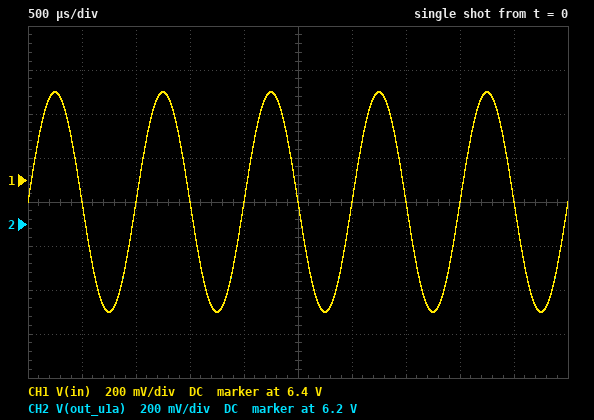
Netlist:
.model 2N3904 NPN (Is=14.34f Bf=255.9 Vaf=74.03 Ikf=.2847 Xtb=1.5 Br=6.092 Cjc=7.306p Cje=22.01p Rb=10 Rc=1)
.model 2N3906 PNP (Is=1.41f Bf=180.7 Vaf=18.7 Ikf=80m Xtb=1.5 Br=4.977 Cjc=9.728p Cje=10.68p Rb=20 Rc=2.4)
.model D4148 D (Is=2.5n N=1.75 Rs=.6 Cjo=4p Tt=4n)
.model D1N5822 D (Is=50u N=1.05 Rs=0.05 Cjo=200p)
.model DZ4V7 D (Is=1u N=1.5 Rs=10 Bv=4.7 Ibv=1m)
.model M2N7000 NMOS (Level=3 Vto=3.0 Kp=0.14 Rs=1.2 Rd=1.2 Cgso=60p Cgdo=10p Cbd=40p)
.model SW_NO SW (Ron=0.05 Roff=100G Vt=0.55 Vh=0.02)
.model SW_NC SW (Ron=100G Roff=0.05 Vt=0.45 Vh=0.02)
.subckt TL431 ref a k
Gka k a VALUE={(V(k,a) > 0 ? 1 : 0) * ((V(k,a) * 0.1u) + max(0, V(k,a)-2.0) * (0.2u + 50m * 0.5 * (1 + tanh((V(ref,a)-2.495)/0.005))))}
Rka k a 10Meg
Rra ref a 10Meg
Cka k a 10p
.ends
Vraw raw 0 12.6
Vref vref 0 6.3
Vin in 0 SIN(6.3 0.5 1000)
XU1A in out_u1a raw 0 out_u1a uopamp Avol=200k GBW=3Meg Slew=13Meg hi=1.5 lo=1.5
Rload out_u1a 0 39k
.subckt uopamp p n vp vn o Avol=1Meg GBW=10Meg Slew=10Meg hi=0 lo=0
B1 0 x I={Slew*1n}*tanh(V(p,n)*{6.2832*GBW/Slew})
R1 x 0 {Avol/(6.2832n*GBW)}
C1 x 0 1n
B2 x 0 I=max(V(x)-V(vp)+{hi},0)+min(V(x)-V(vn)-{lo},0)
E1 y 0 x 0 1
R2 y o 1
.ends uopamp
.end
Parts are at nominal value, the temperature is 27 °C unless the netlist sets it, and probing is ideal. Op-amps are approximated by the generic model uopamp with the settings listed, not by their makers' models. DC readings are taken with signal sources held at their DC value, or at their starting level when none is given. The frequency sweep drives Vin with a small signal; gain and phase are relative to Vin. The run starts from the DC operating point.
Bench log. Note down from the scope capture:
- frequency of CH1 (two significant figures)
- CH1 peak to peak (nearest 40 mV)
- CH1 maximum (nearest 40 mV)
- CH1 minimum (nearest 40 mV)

1.0 kHz
1.00 V
6.80 V
5.80 V
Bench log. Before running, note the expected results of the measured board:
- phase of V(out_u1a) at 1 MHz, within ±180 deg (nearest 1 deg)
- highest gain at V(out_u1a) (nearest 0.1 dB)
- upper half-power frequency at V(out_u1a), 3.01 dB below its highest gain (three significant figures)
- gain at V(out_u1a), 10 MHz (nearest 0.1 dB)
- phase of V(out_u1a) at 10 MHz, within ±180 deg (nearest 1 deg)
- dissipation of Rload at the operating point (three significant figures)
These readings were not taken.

-18 deg
0 dB
3.00 MHz
-10.8 dB
-73 deg
1.02 mW
